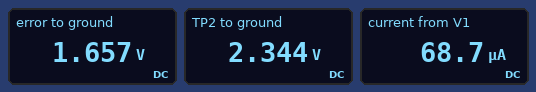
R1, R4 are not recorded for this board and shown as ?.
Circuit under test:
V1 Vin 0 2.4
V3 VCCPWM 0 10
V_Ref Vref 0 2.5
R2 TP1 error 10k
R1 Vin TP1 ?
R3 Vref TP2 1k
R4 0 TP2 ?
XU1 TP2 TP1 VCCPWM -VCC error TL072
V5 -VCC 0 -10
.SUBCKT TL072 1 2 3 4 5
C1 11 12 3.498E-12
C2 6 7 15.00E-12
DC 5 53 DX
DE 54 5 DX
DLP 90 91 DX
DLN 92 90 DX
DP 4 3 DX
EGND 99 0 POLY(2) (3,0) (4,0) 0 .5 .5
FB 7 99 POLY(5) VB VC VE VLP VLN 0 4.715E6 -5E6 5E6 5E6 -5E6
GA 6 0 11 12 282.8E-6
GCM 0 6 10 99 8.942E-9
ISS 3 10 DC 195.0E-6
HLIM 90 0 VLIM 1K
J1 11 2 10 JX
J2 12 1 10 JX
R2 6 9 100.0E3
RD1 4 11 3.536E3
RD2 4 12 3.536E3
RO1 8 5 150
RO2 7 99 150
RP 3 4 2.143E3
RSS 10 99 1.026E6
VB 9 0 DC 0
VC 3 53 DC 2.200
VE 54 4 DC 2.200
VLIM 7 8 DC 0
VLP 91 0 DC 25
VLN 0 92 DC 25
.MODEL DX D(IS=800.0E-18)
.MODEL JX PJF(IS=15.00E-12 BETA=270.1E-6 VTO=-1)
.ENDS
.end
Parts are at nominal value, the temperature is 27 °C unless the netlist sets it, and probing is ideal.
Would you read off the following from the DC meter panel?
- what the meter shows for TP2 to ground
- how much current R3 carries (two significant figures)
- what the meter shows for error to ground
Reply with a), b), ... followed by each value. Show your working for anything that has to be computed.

a) 2.344 V
b) (2.5 V - 2.344 V) / 1 kΩ = 160 µA
c) 1.657 V
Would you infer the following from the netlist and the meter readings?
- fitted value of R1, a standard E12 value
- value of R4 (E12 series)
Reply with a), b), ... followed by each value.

a) 820 Ω
b) 15 kΩ
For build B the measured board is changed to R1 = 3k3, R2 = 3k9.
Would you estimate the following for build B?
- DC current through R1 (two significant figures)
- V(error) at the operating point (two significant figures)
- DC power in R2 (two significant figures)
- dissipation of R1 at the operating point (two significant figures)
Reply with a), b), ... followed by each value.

a) 17 µA
b) 2.3 V
c) 1.1 µW
d) 960 nW
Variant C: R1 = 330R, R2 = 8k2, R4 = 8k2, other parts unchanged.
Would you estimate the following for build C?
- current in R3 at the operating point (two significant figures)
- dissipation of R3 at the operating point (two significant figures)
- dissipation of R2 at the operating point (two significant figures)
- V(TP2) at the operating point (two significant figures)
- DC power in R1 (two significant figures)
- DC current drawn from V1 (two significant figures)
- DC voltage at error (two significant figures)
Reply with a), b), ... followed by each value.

a) 270 µA
b) 74 µW
c) 2.2 mW
d) 2.2 V
e) 89 µW
f) 520 µA
g) -2.0 V
